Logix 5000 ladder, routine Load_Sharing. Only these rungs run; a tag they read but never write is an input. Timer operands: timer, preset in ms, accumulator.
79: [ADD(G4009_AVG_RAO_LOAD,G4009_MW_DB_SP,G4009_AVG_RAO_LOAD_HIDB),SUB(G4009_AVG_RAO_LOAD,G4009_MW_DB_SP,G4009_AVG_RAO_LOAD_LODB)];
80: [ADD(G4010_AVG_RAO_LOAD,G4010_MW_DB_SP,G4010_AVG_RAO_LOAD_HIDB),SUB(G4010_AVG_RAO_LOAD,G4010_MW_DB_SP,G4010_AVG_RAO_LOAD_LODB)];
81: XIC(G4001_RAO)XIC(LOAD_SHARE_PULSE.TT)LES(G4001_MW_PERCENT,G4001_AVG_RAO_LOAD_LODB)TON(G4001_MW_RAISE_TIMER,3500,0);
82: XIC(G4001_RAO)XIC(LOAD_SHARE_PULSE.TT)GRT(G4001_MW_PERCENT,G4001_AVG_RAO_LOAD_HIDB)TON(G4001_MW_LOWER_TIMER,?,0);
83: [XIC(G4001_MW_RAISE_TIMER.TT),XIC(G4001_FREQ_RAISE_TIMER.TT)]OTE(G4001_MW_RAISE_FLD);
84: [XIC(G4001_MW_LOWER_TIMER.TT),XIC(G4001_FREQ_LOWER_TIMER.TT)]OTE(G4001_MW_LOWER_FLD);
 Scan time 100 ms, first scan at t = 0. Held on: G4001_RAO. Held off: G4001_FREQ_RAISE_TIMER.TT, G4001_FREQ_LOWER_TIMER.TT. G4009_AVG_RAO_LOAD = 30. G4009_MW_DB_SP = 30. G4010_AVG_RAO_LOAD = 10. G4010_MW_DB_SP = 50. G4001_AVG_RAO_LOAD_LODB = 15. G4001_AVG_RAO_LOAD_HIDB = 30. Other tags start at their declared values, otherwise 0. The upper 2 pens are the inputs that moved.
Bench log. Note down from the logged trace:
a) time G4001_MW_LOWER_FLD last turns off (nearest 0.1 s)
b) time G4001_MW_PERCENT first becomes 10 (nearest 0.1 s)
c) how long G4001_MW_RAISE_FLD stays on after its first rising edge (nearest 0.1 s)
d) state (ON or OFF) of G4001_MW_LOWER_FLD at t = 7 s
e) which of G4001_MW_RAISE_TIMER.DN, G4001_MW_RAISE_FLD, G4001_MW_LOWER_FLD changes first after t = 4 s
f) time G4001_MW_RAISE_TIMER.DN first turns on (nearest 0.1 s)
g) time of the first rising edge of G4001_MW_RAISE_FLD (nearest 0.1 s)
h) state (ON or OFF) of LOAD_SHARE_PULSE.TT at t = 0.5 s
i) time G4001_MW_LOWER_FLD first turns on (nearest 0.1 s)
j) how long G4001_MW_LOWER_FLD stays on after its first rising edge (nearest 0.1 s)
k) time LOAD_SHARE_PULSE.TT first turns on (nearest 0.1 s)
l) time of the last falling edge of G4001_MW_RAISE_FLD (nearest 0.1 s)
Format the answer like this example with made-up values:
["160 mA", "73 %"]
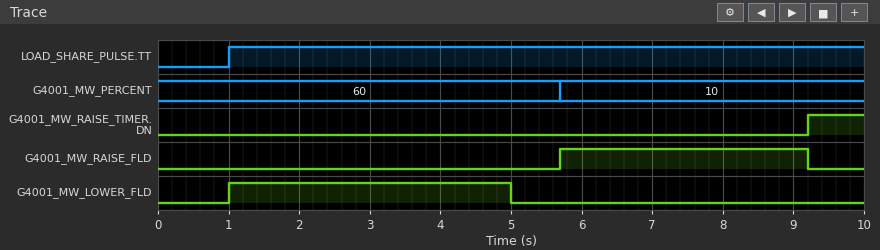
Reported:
["5.0 s", "5.7 s", "3.5 s", "OFF", "G4001_MW_LOWER_FLD", "9.2 s", "5.7 s", "OFF", "1.0 s", "4.0 s", "1.0 s", "9.2 s"]
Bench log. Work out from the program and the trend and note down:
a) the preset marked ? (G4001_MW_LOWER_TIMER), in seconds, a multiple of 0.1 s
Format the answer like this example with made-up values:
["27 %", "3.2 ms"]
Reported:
["4.0 s"]
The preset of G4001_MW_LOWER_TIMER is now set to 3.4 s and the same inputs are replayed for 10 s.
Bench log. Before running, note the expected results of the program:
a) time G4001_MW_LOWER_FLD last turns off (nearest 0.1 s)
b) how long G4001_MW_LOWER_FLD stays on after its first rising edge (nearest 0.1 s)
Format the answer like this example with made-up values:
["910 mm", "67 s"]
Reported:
["4.4 s", "3.4 s"]
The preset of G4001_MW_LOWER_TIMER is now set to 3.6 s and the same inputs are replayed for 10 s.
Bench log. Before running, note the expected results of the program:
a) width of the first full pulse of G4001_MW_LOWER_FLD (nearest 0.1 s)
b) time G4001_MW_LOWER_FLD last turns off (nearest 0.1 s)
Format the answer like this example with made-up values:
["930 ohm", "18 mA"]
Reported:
["3.6 s", "4.6 s"]
